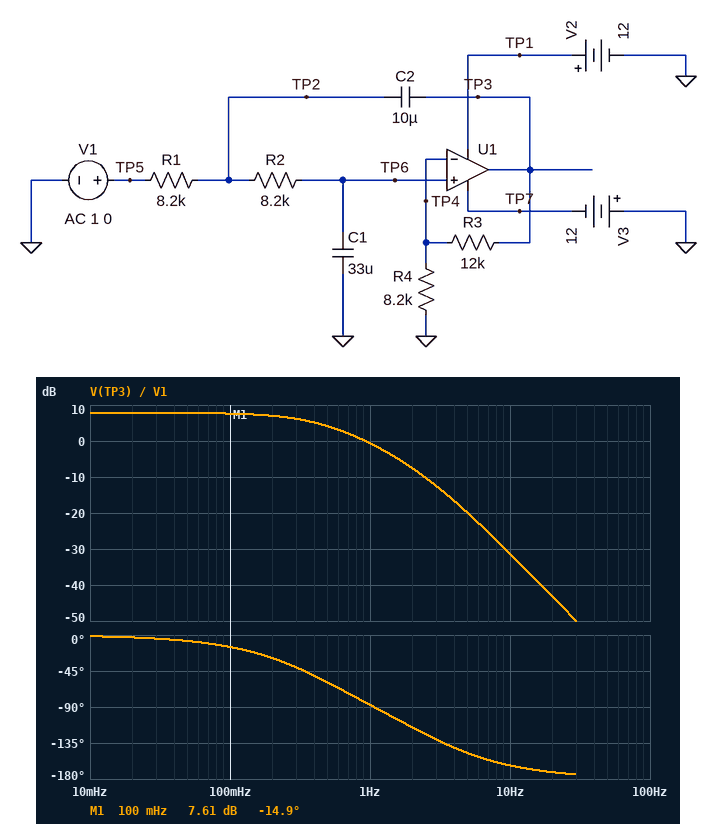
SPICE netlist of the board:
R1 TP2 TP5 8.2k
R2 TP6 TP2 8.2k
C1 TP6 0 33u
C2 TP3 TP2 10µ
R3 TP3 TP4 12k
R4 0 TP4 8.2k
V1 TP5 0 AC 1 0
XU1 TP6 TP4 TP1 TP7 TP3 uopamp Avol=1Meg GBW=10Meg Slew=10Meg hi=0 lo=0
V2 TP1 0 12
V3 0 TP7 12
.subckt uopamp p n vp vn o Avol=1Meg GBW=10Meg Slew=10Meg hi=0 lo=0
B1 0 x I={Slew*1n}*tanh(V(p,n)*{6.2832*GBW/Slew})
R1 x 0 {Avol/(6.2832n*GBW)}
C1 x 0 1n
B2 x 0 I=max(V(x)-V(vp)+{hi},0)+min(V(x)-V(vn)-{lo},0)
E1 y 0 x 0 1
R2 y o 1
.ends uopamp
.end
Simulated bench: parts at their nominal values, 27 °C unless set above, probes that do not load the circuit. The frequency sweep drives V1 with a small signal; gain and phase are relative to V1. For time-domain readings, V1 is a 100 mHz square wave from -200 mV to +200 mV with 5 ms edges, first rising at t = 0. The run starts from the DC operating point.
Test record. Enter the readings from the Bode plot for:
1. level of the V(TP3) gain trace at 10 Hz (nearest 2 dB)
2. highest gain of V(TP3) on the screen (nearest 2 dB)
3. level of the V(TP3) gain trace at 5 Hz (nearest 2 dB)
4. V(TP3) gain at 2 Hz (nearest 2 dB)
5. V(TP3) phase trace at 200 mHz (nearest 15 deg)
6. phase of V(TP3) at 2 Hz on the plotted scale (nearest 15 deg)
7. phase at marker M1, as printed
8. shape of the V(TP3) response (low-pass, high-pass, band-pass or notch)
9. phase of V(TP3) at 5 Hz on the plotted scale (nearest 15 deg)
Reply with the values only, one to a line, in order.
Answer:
-32 dB
8 dB
-20 dB
-8 dB
-30 deg
-120 deg
-14.9 deg
low-pass
-150 deg
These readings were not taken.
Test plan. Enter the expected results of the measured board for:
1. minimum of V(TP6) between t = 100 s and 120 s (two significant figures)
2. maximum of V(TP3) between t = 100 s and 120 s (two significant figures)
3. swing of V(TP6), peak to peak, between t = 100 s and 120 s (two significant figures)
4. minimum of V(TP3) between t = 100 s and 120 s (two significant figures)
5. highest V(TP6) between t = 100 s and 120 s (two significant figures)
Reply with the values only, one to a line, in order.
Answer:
-200 mV
490 mV
400 mV
-490 mV
200 mV
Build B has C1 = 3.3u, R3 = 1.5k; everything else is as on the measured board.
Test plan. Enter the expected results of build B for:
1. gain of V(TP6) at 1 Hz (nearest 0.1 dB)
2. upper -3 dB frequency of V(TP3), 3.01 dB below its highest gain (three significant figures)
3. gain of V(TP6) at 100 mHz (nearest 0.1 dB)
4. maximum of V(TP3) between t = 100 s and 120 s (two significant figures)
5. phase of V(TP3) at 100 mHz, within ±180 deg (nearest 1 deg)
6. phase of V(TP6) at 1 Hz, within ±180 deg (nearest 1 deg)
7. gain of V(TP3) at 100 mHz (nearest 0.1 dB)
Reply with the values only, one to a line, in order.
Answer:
0.5 dB
4.01 Hz
0 dB
350 mV
-1 deg
-15 deg
1.5 dB
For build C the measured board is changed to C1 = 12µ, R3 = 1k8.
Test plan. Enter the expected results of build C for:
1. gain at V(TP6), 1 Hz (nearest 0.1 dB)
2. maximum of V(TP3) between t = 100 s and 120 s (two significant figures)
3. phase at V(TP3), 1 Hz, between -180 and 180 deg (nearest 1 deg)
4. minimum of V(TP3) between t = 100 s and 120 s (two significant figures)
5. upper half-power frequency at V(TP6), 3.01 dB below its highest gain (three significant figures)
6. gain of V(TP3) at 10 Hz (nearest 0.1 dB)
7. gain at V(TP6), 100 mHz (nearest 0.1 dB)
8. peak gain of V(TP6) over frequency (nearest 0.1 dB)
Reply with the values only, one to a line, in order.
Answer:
-2.4 dB
240 mV
-59 deg
-240 mV
1.15 Hz
-28.6 dB
0 dB
0 dB
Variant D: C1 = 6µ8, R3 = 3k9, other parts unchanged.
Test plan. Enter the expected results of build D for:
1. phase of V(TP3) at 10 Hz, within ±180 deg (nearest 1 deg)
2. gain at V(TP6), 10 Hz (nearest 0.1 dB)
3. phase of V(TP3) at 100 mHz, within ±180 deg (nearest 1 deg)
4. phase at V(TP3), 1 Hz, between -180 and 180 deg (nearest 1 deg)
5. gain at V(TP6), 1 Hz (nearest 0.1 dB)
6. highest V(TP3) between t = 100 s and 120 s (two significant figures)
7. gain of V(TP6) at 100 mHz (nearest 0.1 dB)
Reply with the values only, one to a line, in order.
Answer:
-165 deg
-24.9 dB
-3 deg
-29 deg
0.6 dB
380 mV
0 dB
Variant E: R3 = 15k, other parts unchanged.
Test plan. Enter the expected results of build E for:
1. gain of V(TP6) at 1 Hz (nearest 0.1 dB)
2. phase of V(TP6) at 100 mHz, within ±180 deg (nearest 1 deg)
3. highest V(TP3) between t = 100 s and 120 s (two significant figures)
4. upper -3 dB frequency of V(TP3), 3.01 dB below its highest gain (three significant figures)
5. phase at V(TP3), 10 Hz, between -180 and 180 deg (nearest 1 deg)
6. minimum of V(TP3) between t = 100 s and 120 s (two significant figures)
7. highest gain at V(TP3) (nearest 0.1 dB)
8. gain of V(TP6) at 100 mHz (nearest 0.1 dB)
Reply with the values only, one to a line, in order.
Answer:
-7.8 dB
-14 deg
570 mV
473 mHz
-164 deg
-570 mV
9.0 dB
-0.2 dB
